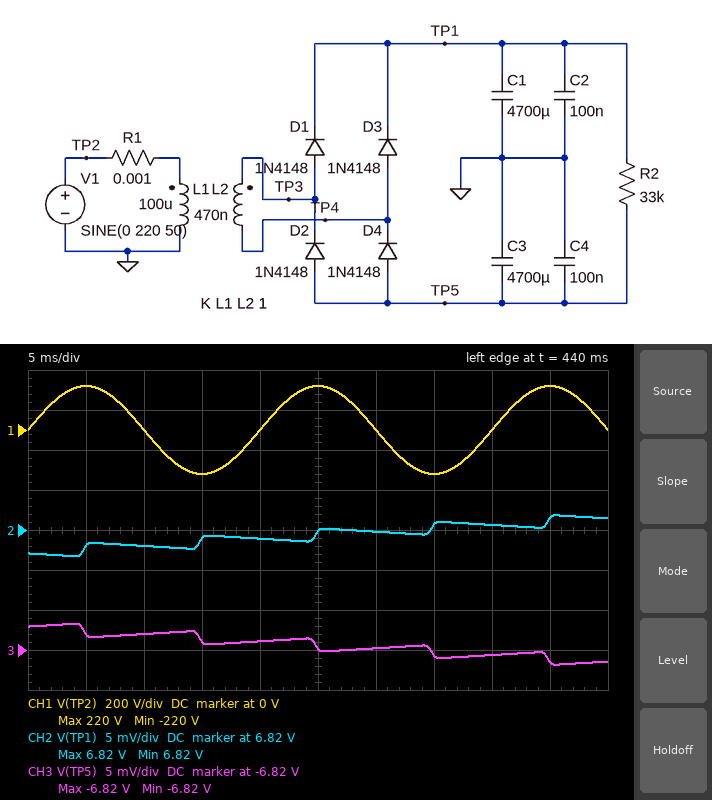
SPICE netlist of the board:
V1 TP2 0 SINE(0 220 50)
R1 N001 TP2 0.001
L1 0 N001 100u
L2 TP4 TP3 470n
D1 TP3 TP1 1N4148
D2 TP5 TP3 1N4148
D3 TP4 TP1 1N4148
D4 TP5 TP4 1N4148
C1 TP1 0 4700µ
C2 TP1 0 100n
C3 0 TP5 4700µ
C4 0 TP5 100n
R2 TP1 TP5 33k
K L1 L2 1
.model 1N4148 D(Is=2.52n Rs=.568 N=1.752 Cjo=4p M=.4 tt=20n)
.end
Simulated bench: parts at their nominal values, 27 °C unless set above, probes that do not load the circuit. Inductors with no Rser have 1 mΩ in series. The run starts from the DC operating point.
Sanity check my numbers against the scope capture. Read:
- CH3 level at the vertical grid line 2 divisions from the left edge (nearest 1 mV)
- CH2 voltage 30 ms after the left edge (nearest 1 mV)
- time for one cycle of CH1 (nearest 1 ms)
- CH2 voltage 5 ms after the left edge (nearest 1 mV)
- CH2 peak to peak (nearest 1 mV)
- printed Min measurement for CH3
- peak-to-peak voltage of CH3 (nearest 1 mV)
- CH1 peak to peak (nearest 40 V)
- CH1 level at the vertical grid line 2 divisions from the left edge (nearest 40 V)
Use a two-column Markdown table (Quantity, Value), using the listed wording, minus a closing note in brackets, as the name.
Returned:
| Quantity | Value |
|---|---|
| CH3 level at the vertical grid line 2 divisions from the left edge | -6.818 V |
| CH2 voltage 30 ms after the left edge | 6.820 V |
| time for one cycle of CH1 | 20 ms |
| CH2 voltage 5 ms after the left edge | 6.818 V |
| CH2 peak to peak | 5 mV |
| printed Min measurement for CH3 | -6.82 V |
| peak-to-peak voltage of CH3 | 5 mV |
| CH1 peak to peak | 440 V |
| CH1 level at the vertical grid line 2 divisions from the left edge | 0 V |
